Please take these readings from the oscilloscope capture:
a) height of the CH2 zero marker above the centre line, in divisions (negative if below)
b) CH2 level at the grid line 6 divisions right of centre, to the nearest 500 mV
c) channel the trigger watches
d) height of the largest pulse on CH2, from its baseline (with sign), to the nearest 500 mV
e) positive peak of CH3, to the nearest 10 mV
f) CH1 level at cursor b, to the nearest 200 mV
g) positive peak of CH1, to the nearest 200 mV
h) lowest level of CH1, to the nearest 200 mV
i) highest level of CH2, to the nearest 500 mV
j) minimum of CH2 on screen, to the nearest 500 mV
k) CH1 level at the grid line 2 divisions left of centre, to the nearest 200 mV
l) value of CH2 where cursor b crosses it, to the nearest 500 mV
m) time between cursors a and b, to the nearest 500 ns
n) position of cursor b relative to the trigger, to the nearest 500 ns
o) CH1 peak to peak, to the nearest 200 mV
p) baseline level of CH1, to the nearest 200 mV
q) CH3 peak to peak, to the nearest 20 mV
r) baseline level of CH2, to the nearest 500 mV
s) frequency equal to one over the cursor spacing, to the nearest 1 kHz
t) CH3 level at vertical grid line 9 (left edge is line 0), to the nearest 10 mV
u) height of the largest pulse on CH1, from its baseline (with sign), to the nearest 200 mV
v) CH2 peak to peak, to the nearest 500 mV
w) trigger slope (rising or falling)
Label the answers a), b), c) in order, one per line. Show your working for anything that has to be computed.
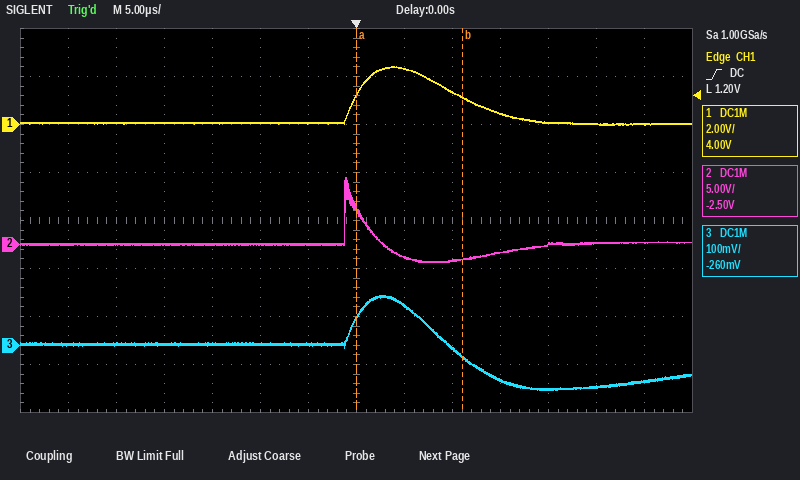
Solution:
a) -0.5 div
b) 0.0 V
c) CH1
d) 7.0 V − (0.0 V) = +7.0 V
e) 100 mV
f) 1.2 V
g) 2.4 V
h) 0.0 V
i) 7.0 V
j) -2.0 V
k) 0.0 V
l) -1.5 V
m) 11.0 µs
n) +11.0 µs
o) 2.4 V − (0.0 V) = 2.4 V
p) 0.0 V
q) 200 mV
r) 0.0 V
s) 1 / 11.0 µs ≈ 91 kHz
t) -10 mV
u) 2.4 V − (0.0 V) = +2.4 V
v) 7.0 V − (-2.0 V) = 9.0 V
w) rising
